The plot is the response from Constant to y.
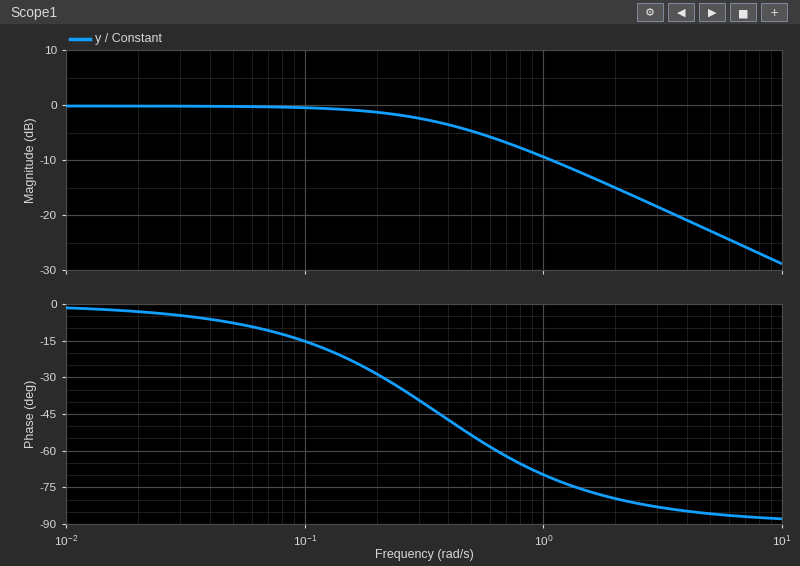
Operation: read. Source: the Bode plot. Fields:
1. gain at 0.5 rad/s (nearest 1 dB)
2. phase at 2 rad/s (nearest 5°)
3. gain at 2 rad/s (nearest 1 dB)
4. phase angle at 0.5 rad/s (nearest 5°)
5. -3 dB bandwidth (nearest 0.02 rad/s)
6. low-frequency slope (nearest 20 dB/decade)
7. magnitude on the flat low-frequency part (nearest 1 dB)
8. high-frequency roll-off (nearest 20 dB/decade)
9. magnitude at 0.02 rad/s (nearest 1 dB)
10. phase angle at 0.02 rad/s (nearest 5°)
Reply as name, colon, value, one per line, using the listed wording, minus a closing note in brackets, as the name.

gain at 0.5 rad/s: -5 dB
phase at 2 rad/s: -80°
gain at 2 rad/s: -15 dB
phase angle at 0.5 rad/s: -55°
-3 dB bandwidth: 0.36 rad/s
low-frequency slope: 0 dB/decade
magnitude on the flat low-frequency part: 0 dB
high-frequency roll-off: -20 dB/decade
magnitude at 0.02 rad/s: 0 dB
phase angle at 0.02 rad/s: -5°
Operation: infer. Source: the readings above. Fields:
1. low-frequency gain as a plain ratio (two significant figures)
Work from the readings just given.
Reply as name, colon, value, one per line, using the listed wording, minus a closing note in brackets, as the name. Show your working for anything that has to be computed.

low-frequency gain as a plain ratio: 10^(0 / 20) = 1.0
